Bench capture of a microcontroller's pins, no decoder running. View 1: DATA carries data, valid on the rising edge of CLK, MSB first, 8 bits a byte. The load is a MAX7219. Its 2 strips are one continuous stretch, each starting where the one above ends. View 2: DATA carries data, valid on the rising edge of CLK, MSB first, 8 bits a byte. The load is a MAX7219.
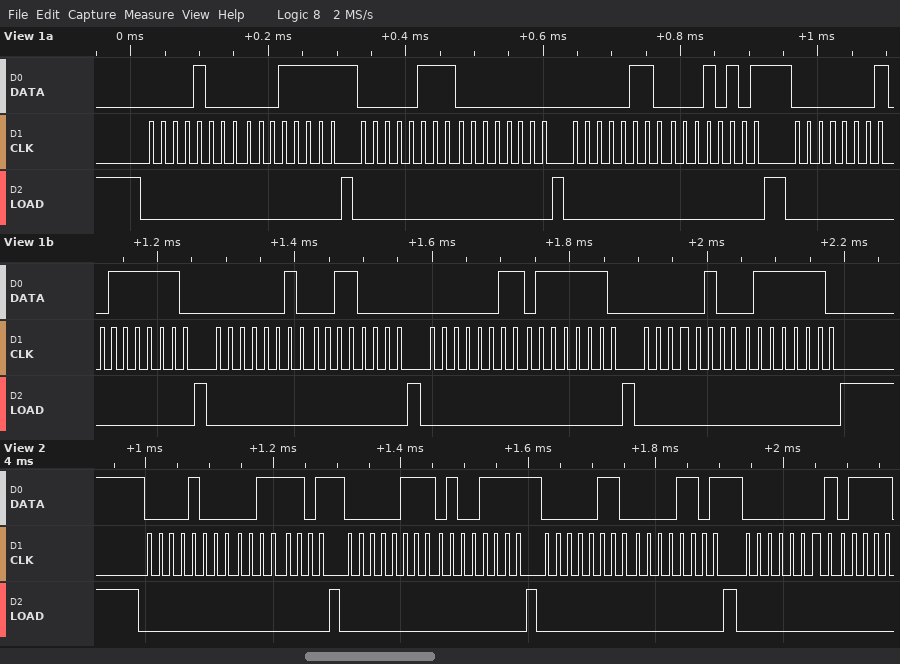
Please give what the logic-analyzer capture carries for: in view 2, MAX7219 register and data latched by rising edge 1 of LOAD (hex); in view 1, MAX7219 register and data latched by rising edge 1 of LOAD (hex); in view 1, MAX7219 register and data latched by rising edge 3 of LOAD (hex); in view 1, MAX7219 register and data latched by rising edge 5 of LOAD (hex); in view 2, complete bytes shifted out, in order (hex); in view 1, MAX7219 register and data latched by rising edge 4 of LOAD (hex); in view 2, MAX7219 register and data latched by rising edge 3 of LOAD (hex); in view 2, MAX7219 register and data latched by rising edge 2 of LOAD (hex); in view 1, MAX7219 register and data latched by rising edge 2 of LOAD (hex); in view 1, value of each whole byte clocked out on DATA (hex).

register 0x8, data 0x3D
register 0x8, data 0x1F
register 0x6, data 0x15
register 0x2, data 0x30
08 3D 07 4F 06 0D 01
register 0x1, data 0x7E
register 0x6, data 0x0D
register 0x7, data 0x4F
register 0x7, data 0x00
0x08 0x1F 0x07 0x00 0x06 0x15 0x01 0x7E 0x02 0x30 0x03 0x7E 0x04 0x7E
